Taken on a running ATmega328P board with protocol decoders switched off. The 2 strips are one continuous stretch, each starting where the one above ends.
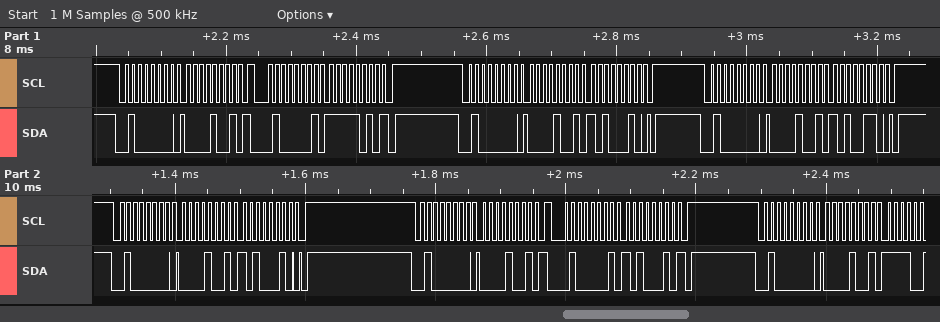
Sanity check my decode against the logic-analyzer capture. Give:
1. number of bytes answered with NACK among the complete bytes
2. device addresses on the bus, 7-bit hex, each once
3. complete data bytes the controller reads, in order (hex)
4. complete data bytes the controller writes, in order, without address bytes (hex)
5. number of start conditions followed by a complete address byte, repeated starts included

2
0x20
FA A2
09 09 A2 09 A6 09 A2 09 09
8
